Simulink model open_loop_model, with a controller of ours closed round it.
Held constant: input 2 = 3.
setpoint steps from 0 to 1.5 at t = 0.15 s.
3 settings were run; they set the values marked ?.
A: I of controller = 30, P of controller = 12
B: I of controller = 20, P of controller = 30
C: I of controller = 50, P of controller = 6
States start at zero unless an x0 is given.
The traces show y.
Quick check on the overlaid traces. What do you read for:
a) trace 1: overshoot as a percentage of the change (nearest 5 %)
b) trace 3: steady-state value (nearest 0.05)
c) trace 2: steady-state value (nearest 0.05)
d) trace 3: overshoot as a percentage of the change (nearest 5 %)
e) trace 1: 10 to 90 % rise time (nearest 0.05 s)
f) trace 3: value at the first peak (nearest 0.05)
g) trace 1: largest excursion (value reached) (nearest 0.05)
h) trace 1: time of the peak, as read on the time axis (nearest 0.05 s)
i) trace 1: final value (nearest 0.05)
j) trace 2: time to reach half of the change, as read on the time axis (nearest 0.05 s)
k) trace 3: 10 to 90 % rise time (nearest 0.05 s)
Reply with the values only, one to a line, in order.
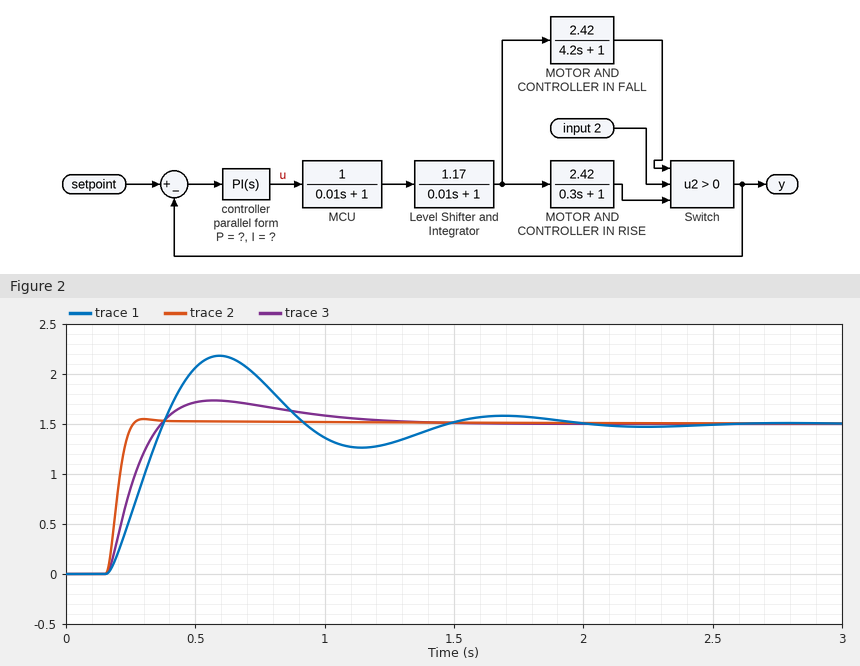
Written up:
45 %
1.50
1.50
15 %
0.15 s
1.75
2.20
0.60 s
1.50
0.20 s
0.15 s
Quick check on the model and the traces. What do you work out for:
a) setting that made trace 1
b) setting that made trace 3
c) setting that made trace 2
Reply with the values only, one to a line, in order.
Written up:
C
A
B
